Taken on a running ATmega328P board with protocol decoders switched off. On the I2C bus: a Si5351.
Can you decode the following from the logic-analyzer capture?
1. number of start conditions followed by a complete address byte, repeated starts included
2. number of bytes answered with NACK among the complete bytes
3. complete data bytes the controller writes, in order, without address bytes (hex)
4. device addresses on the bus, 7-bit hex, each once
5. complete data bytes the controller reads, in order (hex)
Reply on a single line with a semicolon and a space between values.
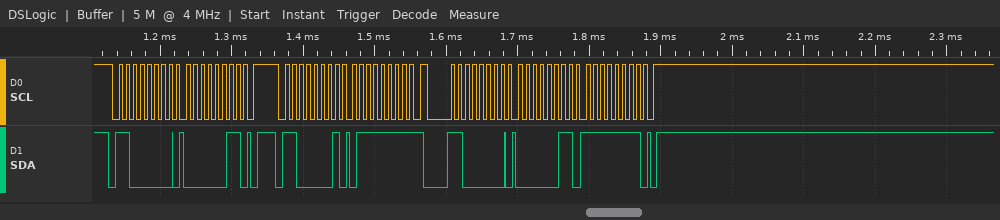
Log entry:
3; 1; 03 03 FF; 0x60; 7F
